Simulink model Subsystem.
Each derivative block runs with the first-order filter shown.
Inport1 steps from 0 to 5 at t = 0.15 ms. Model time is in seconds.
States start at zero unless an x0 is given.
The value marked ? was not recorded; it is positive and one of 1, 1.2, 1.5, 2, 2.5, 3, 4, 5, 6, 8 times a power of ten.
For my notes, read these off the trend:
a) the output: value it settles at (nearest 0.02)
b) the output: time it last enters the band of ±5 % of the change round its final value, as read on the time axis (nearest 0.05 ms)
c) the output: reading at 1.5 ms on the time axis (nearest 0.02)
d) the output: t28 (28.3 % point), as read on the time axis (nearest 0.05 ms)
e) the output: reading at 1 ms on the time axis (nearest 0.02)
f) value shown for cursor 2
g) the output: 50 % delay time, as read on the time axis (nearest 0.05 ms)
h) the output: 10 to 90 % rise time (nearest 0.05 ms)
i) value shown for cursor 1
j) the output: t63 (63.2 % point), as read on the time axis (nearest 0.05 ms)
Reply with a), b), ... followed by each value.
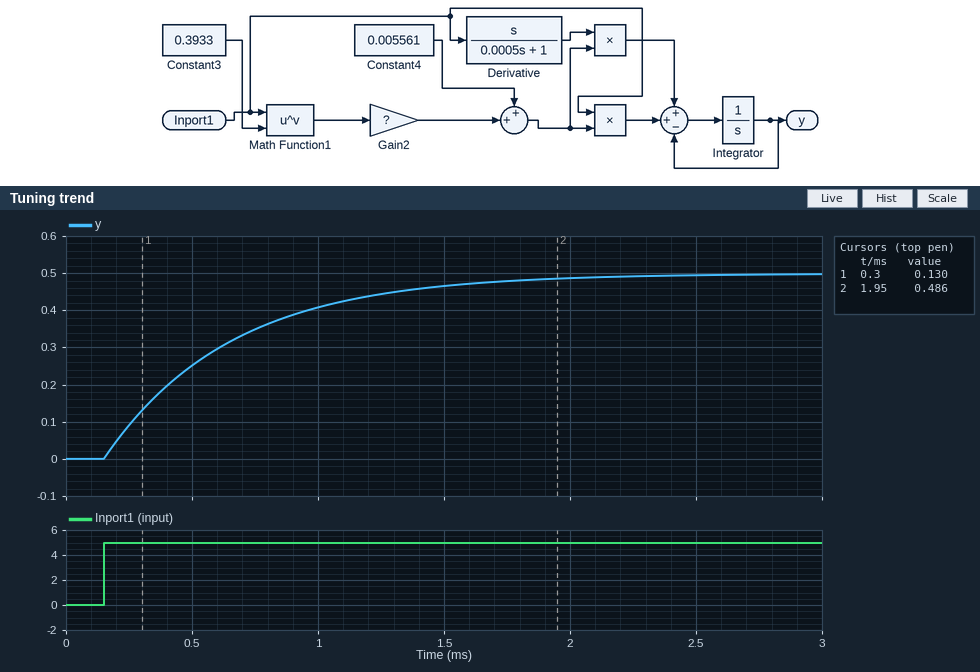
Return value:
a) 0.50
b) 1.65 ms
c) 0.46
d) 0.30 ms
e) 0.40
f) 0.486
g) 0.50 ms
h) 1.10 ms
i) 0.130
j) 0.65 ms
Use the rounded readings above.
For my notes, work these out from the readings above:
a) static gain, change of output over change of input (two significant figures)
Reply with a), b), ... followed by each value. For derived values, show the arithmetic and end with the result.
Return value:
a) (0.5 - 0) / (5 - 0) = 0.10
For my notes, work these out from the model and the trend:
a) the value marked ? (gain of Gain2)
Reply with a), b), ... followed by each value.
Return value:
a) 0.05
